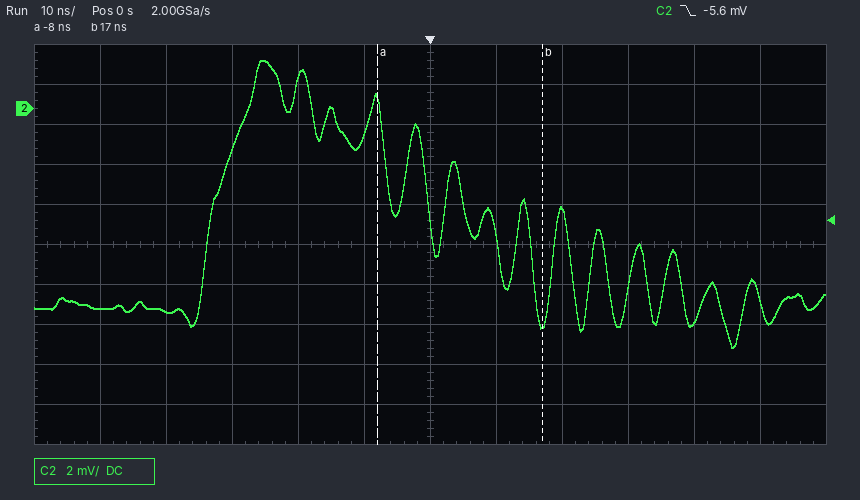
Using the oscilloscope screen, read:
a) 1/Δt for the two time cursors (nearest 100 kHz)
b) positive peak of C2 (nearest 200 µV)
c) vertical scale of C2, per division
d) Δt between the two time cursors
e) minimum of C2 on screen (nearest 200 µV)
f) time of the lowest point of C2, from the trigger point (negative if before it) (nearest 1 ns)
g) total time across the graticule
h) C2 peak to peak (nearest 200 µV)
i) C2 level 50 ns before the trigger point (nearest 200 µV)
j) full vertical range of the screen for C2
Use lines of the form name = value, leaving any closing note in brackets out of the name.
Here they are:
1/Δt for the two time cursors = 40.0 MHz
positive peak of C2 = 2.4 mV
vertical scale of C2, per division = 2 mV
Δt between the two time cursors = 25 ns
minimum of C2 on screen = -12.0 mV
time of the lowest point of C2, from the trigger point (negative if before it) = +46 ns
total time across the graticule = 120 ns
C2 peak to peak = 14.4 mV
C2 level 50 ns before the trigger point = -10.0 mV
full vertical range of the screen for C2 = 20 mV
